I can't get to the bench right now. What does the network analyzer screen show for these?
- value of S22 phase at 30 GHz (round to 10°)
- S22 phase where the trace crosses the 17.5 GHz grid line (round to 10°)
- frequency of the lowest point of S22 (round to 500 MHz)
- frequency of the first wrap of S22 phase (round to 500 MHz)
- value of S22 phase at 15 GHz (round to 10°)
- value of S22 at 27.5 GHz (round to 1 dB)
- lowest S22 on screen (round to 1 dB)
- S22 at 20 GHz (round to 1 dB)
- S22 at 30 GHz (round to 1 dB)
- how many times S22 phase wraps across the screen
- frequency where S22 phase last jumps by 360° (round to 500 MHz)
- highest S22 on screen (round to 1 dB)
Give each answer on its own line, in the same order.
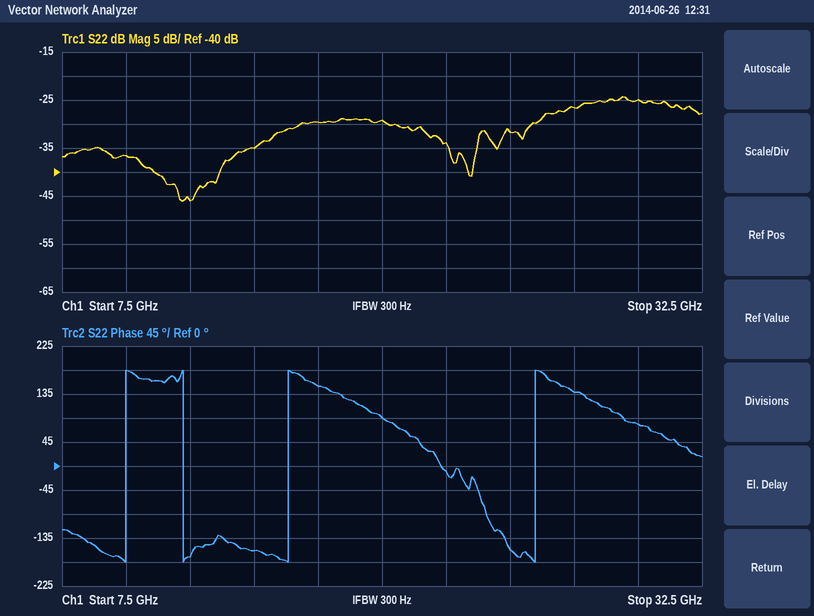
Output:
80°
150°
12.0 GHz
10.0 GHz
-160°
-27 dB
-46 dB
-29 dB
-25 dB
4
26.0 GHz
-24 dB
